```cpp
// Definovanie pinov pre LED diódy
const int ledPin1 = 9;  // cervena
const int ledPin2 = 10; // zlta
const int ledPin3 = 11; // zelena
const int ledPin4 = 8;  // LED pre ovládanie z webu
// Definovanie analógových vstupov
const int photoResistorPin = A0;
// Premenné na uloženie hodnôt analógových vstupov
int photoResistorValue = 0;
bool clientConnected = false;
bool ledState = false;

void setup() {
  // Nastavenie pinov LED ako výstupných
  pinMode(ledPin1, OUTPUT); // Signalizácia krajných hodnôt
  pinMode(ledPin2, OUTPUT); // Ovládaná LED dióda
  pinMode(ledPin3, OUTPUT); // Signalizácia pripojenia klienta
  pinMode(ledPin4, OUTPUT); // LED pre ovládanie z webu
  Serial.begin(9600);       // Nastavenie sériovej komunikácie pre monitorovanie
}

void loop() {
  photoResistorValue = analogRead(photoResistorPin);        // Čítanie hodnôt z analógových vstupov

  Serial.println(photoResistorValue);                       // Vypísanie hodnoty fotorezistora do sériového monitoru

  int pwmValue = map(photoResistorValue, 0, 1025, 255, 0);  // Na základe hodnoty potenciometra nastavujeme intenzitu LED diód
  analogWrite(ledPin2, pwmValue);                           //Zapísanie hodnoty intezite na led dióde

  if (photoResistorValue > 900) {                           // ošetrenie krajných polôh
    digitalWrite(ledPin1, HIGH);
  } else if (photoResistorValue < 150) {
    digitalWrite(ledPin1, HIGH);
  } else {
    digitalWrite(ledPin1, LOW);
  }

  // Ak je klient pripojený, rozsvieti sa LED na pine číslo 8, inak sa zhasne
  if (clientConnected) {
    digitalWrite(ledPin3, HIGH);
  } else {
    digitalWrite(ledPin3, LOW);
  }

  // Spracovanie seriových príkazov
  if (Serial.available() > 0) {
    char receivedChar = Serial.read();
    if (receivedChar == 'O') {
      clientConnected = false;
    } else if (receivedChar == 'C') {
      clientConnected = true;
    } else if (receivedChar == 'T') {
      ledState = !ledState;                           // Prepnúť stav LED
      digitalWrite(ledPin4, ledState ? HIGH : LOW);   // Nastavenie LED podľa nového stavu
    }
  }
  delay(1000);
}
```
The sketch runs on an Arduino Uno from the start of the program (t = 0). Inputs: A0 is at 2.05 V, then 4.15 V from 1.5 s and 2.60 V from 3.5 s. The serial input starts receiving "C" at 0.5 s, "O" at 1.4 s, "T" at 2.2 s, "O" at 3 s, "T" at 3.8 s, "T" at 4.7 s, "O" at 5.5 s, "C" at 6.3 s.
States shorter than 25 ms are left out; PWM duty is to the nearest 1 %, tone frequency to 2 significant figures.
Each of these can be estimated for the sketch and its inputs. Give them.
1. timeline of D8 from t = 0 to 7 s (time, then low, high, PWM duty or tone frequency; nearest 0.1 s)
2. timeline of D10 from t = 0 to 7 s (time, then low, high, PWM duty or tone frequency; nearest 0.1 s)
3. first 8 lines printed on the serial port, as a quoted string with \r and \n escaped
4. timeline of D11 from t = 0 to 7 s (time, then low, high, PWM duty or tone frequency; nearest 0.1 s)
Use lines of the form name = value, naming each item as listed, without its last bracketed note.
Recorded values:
timeline of D8 from t = 0 to 7 s = 0 s low; 3 s high; 5 s low; 6 s high
timeline of D10 from t = 0 to 7 s = 0 s PWM 59 %; 2 s PWM 17 %; 4 s PWM 48 %
first 8 lines printed on the serial port, as a quoted string with \r and \n escaped = "419\r\n419\r\n849\r\n849\r\n532\r\n532\r\n532\r\n532\r\n"
timeline of D11 from t = 0 to 7 s = 0 s low; 2 s high; 3 s low
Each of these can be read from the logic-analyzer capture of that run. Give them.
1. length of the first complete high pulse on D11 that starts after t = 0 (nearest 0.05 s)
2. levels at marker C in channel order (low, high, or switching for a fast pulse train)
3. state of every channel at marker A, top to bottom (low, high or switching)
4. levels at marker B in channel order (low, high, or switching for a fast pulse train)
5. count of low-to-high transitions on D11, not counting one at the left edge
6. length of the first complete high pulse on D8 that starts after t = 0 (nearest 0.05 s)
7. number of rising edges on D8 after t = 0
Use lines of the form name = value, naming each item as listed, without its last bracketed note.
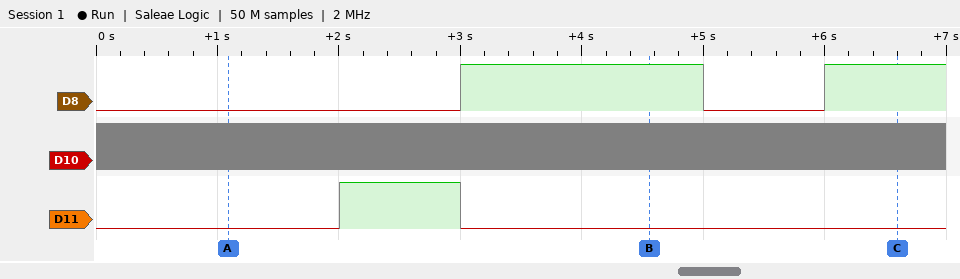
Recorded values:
length of the first complete high pulse on D11 that starts after t = 0 = 1.00 s
levels at marker C in channel order = D8 high, D10 switching, D11 low
state of every channel at marker A, top to bottom = D8 low, D10 switching, D11 low
levels at marker B in channel order = D8 high, D10 switching, D11 low
count of low-to-high transitions on D11, not counting one at the left edge = 1
length of the first complete high pulse on D8 that starts after t = 0 = 2.00 s
number of rising edges on D8 after t = 0 = 2
